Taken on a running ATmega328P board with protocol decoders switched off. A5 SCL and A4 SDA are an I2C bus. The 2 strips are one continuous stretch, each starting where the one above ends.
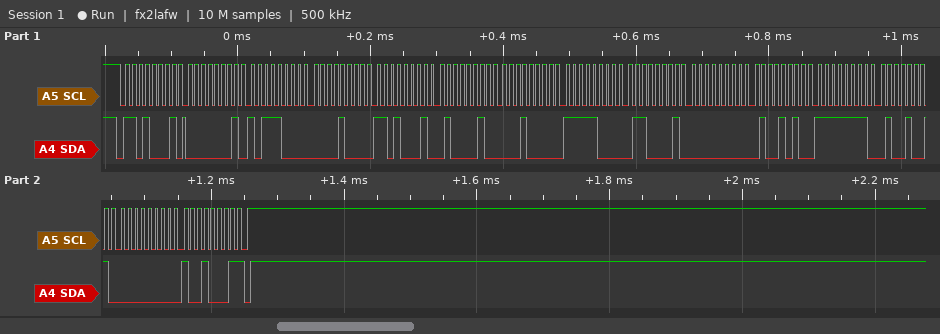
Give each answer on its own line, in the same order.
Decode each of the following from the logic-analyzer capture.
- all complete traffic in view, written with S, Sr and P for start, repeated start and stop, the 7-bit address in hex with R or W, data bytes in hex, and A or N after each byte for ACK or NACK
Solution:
S 68R A 01 A B8 A 08 A D1 A 42 A 10 A F8 A 61 A 00 A 4A A FF A 49 A 00 A 91 N P
